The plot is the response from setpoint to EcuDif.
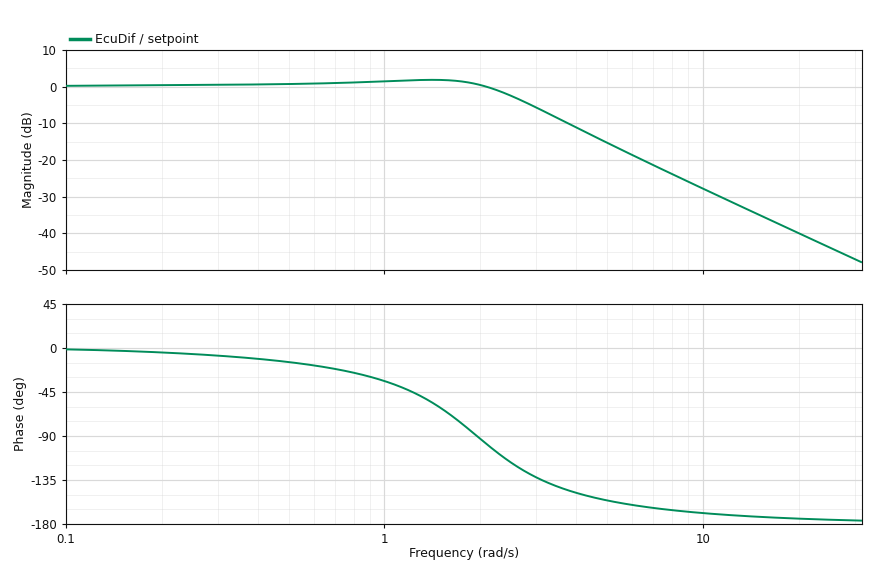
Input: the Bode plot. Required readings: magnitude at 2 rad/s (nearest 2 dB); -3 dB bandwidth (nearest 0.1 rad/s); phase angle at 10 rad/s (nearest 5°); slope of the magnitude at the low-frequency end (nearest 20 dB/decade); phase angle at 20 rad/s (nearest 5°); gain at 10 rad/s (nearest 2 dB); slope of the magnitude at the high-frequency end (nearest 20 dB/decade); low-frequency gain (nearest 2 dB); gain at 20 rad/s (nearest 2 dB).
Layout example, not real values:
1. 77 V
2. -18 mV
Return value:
1. 0 dB
2. 2.5 rad/s
3. -170°
4. 0 dB/decade
5. -175°
6. -28 dB
7. -40 dB/decade
8. 0 dB
9. -40 dB
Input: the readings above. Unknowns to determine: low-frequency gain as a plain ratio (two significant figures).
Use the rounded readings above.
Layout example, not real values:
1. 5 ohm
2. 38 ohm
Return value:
1. 1.0
